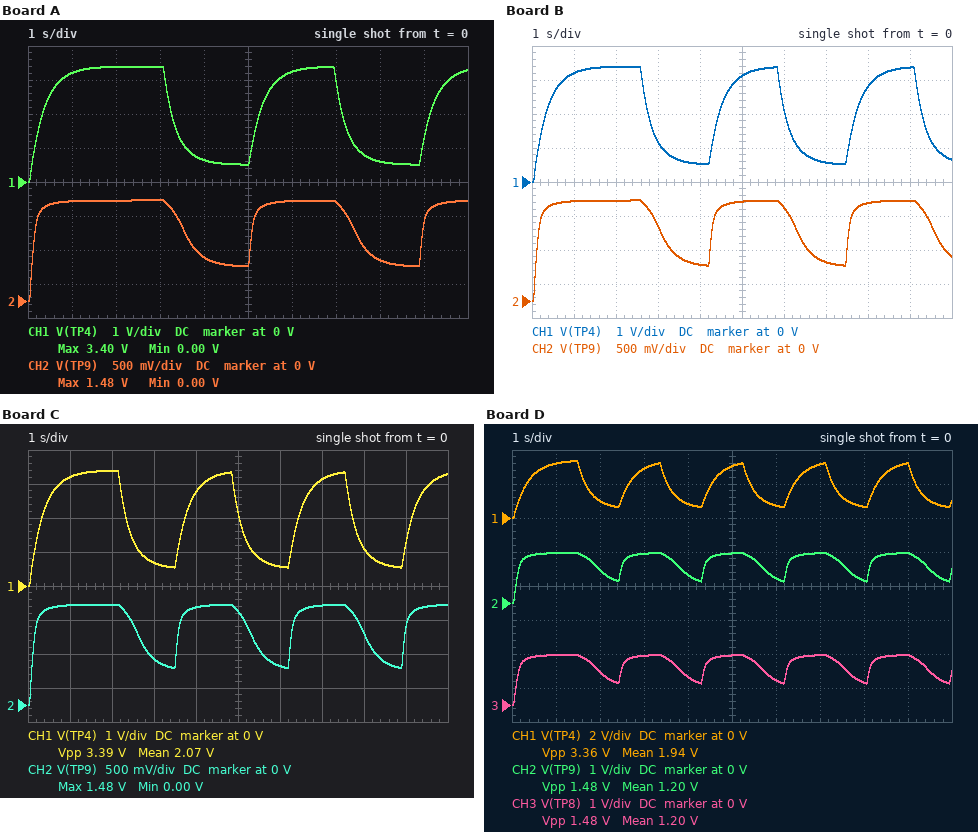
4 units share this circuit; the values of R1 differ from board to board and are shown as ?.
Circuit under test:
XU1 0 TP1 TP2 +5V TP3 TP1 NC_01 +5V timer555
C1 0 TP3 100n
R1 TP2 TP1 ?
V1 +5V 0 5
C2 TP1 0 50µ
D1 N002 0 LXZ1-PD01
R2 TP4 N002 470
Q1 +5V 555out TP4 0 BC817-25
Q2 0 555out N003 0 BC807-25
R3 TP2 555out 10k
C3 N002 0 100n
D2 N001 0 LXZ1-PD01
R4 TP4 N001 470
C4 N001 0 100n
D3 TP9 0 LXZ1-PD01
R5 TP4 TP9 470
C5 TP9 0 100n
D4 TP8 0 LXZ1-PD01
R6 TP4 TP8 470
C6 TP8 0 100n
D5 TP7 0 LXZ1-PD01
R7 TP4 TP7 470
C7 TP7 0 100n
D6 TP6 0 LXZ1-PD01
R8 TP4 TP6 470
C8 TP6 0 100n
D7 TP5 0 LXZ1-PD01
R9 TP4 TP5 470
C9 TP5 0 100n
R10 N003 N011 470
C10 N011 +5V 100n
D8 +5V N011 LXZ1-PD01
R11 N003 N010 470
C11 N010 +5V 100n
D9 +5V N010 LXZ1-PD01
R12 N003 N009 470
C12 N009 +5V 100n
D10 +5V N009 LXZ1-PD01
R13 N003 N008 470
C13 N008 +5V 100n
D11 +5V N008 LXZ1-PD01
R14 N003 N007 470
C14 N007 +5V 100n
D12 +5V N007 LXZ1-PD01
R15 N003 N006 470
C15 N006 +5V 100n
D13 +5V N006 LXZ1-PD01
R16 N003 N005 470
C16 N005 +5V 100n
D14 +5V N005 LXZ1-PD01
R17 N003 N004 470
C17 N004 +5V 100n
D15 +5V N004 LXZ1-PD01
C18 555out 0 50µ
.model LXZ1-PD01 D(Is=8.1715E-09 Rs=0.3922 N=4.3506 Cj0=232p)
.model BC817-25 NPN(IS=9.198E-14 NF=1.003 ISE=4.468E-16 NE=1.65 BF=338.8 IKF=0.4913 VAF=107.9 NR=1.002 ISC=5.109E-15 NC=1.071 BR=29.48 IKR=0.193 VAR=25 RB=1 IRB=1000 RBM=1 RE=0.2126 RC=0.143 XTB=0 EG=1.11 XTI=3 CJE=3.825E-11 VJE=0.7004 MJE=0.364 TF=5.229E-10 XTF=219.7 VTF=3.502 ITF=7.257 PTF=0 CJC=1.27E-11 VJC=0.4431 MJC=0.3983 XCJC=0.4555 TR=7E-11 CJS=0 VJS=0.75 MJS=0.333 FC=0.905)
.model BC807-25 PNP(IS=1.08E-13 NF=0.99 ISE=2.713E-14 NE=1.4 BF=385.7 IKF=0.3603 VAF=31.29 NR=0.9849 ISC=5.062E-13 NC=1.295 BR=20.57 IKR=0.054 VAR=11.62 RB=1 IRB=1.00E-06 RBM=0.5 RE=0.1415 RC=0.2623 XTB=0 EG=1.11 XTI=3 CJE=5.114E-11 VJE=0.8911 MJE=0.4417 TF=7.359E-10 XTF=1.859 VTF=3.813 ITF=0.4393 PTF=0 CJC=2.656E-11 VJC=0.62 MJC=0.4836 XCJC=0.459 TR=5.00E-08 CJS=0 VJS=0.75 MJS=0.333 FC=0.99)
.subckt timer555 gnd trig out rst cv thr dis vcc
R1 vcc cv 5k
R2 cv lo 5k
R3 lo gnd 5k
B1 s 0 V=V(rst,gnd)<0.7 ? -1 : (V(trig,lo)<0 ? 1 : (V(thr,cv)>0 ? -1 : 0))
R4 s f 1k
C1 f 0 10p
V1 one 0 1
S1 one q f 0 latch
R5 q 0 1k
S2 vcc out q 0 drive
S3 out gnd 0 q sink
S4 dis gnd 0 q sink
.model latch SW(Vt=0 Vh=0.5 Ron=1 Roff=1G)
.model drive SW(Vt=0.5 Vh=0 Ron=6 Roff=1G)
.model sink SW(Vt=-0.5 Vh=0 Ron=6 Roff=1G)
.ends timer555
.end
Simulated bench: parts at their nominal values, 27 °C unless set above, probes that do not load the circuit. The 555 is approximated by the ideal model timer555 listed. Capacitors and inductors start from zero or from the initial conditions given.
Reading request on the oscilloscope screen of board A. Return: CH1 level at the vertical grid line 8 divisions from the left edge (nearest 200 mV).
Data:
600 mV
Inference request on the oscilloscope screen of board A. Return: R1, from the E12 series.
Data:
56 kΩ
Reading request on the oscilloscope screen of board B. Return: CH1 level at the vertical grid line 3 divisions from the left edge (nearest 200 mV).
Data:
1.2 V
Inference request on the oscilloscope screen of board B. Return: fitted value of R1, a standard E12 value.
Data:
47 kΩ
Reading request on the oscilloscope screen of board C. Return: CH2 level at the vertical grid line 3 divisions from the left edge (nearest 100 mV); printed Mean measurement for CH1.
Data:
700 mV
2.07 V
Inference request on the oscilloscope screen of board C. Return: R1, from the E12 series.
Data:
39 kΩ
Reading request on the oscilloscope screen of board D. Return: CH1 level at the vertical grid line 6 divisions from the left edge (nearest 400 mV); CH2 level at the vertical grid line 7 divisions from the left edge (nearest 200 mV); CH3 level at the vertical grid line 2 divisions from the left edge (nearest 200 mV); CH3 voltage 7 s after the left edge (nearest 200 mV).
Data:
800 mV
1.4 V
1.0 V
1.4 V
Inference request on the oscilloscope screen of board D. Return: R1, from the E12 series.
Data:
27 kΩ
